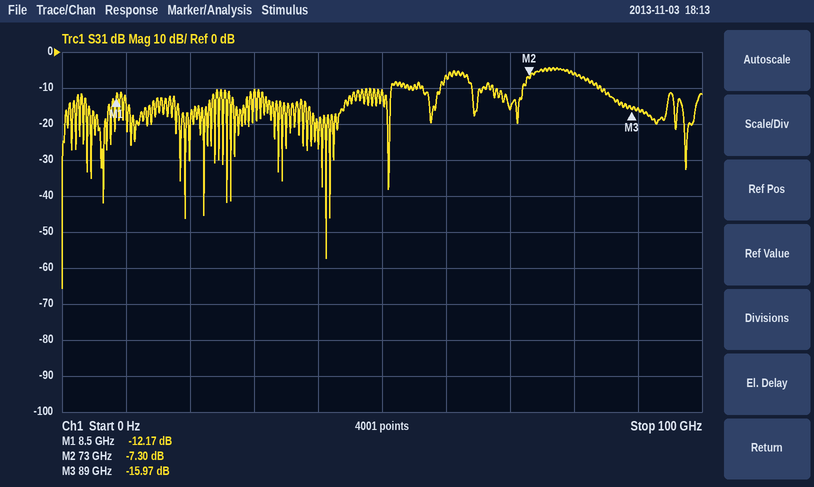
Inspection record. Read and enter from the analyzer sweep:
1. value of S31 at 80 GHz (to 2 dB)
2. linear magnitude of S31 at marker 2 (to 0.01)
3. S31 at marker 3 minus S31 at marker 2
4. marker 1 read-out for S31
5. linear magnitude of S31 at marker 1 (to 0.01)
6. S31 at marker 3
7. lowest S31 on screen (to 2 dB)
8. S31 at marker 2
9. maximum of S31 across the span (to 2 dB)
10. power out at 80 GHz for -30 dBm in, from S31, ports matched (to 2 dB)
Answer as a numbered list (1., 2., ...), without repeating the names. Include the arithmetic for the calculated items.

1. -6 dB
2. 10^(-7.3/20) ≈ 0.43
3. -15.97 − (-7.3) = -8.67 dB
4. -12.17 dB
5. 10^(-12.17/20) ≈ 0.25
6. -15.97 dB
7. -66 dB
8. -7.30 dB
9. -4 dB
10. -30 dBm + (-6 dB) = -36 dBm
